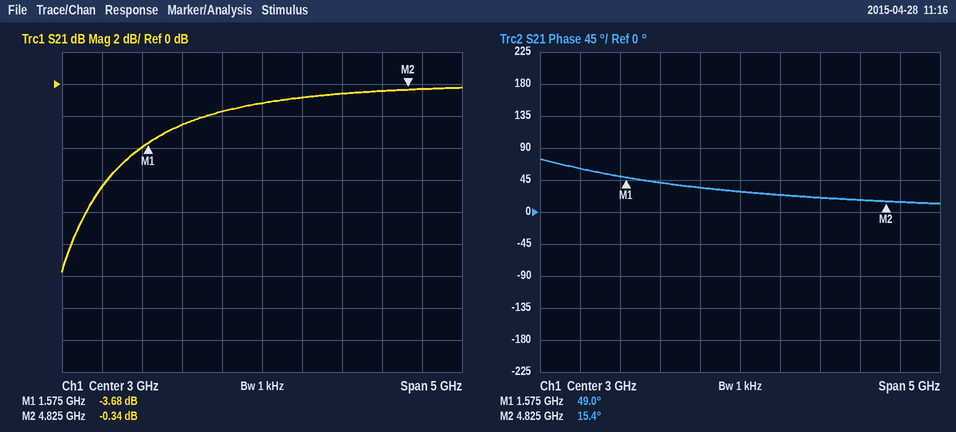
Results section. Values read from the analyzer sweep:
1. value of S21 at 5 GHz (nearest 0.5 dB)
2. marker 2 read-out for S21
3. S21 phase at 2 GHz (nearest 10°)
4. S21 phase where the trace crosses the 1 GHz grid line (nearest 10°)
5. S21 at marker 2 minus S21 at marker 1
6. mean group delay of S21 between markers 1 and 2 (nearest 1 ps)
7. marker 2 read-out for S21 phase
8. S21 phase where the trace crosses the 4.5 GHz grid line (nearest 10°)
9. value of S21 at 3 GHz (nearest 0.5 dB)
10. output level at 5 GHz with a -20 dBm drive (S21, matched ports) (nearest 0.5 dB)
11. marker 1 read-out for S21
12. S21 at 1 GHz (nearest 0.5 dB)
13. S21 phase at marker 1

-0.5 dB
-0.34 dB
40°
60°
3.34 dB
29 ps
15.4°
20°
-1.0 dB
-20.5 dBm
-3.68 dB
-6.5 dB
49.0°
